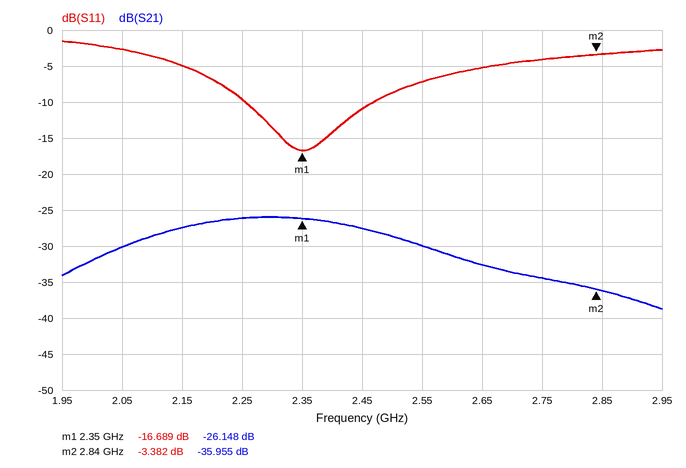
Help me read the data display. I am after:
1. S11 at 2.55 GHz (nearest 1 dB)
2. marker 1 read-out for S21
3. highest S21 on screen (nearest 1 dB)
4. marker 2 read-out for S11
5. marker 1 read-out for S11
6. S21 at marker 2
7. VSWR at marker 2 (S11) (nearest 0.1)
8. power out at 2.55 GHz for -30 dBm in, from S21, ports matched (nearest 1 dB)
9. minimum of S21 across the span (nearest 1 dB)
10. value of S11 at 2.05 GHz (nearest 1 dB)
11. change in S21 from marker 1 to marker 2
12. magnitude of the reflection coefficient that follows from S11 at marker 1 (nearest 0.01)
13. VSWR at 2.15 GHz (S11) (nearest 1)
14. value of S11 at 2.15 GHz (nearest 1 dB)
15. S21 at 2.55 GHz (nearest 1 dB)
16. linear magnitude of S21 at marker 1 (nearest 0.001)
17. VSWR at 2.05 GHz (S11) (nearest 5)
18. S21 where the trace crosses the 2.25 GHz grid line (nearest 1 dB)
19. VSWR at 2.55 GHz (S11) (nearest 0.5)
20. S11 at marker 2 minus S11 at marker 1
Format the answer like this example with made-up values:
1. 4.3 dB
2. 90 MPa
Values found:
1. -7 dB
2. -26.148 dB
3. -26 dB
4. -3.382 dB
5. -16.689 dB
6. -35.955 dB
7. 5.2
8. -60 dBm
9. -39 dB
10. -3 dB
11. -9.807 dB
12. 0.15
13. 4
14. -5 dB
15. -30 dB
16. 0.049
17. 5
18. -26 dB
19. 2.5
20. 13.307 dB
